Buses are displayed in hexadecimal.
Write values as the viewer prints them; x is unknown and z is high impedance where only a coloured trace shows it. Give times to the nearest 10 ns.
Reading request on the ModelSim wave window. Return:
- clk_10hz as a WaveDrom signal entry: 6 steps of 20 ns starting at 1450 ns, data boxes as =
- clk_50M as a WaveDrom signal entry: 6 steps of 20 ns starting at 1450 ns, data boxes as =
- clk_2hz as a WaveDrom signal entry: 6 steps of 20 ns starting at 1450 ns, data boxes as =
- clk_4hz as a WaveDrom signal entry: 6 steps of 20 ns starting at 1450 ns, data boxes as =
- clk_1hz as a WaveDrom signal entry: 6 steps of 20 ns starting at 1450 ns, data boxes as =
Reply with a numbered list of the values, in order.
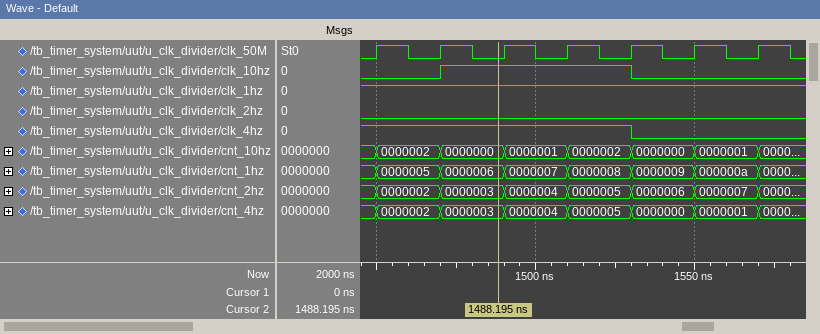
1. {name: 'clk_10hz', wave: '01..0.'}
2. {name: 'clk_50M', wave: 'p.....'}
3. {name: 'clk_2hz', wave: '0.....'}
4. {name: 'clk_4hz', wave: '1...0.'}
5. {name: 'clk_1hz', wave: '1.....'}
